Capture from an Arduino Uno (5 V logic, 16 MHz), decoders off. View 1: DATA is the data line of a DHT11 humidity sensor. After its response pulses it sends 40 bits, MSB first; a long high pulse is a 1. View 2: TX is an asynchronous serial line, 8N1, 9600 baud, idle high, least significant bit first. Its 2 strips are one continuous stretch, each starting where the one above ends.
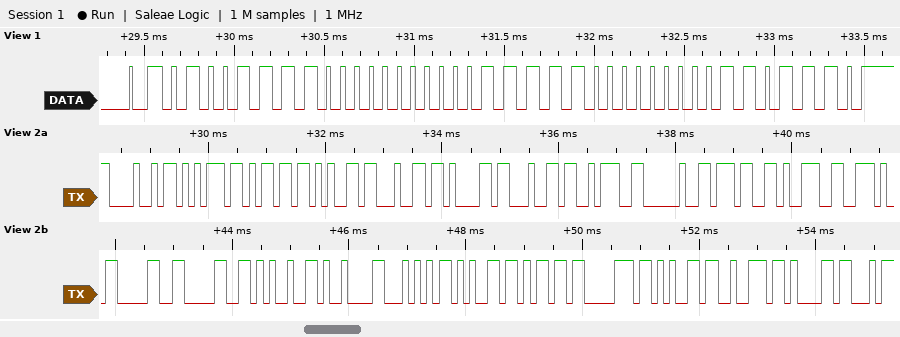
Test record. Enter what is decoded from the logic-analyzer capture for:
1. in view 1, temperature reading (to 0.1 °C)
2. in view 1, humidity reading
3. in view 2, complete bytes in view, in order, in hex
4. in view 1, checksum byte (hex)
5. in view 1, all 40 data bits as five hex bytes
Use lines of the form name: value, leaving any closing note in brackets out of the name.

in view 1, temperature reading: 31.0 °C
in view 1, humidity reading: 79 %
in view 2, complete bytes in view, in order, in hex: 48 75 6D 65 64 61 64 3A 20 37 39 2E 30 30 25 09 54 65 6D 70 65 72 61
in view 1, checksum byte: 0x6E
in view 1, all 40 data bits as five hex bytes: 4F 00 1F 00 6E
